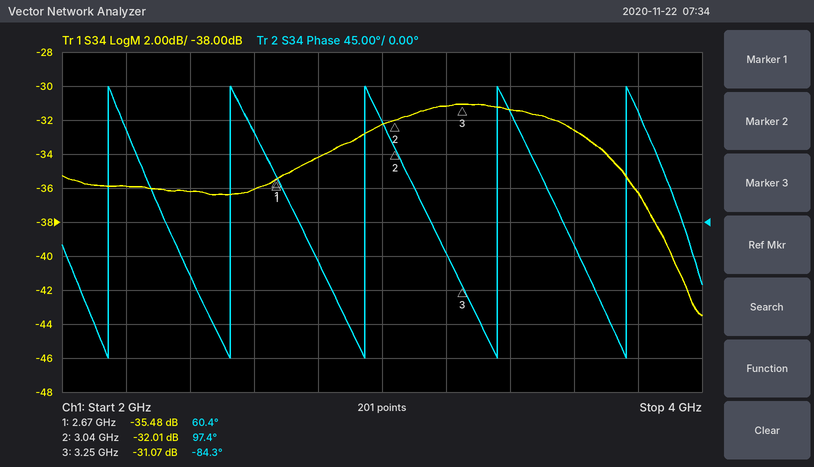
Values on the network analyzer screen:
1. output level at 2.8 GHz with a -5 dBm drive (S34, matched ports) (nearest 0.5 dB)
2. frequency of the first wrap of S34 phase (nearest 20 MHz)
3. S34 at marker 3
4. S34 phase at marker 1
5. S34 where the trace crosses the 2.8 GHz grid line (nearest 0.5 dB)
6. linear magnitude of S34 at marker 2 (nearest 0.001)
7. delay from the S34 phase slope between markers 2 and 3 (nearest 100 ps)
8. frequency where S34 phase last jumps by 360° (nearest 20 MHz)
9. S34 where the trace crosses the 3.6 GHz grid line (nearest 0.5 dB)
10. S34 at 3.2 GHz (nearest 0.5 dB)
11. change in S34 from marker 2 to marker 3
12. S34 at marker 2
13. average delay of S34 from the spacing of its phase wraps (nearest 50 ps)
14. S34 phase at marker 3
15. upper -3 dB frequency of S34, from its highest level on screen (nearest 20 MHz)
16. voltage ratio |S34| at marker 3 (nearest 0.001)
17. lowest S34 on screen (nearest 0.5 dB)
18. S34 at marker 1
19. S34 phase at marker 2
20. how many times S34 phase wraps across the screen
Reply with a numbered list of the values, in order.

1. -39.0 dBm
2. 2.14 GHz
3. -31.07 dB
4. 60.4°
5. -34.0 dB
6. 0.025
7. 2.4 ns
8. 3.76 GHz
9. -32.5 dB
10. -31.0 dB
11. 0.94 dB
12. -32.01 dB
13. 2.45 ns
14. -84.3°
15. 3.70 GHz
16. 0.028
17. -43.5 dB
18. -35.48 dB
19. 97.4°
20. 5
